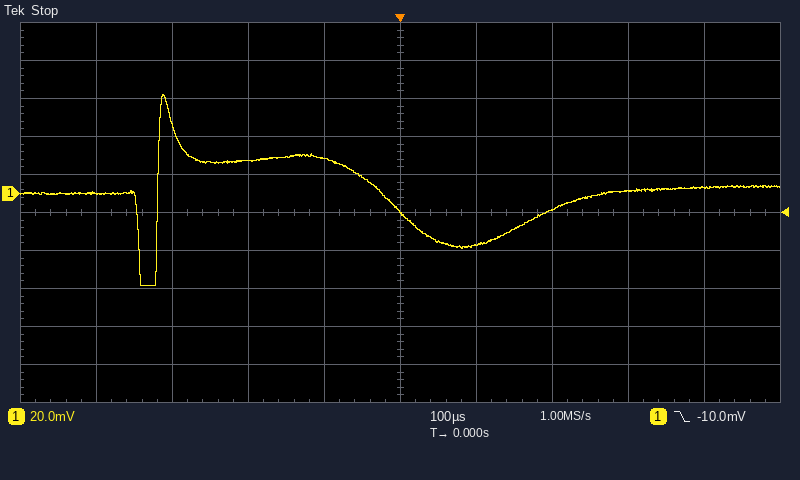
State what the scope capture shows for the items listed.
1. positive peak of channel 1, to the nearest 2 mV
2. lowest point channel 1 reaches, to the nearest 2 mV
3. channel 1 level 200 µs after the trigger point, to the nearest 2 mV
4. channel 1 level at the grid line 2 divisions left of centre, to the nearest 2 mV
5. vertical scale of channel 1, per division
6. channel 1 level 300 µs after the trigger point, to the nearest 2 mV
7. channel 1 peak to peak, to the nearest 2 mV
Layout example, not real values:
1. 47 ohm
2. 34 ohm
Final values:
1. 52 mV
2. -48 mV
3. -8 mV
4. 18 mV
5. 20 mV
6. 2 mV
7. 100 mV
